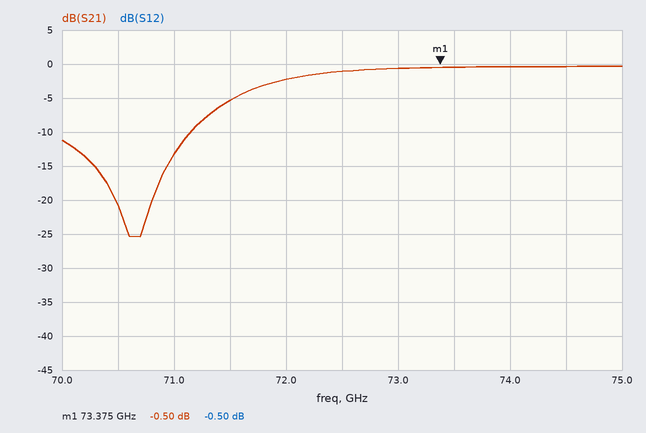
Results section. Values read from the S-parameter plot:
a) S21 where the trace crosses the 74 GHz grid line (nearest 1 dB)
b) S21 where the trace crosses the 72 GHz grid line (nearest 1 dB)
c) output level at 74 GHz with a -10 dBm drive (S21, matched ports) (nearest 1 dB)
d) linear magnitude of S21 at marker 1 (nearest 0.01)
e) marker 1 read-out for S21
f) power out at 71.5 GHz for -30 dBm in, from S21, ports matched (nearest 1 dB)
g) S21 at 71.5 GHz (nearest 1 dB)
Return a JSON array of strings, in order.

["0 dB", "-2 dB", "-10 dBm", "0.94", "-0.50 dB", "-35 dBm", "-5 dB"]
